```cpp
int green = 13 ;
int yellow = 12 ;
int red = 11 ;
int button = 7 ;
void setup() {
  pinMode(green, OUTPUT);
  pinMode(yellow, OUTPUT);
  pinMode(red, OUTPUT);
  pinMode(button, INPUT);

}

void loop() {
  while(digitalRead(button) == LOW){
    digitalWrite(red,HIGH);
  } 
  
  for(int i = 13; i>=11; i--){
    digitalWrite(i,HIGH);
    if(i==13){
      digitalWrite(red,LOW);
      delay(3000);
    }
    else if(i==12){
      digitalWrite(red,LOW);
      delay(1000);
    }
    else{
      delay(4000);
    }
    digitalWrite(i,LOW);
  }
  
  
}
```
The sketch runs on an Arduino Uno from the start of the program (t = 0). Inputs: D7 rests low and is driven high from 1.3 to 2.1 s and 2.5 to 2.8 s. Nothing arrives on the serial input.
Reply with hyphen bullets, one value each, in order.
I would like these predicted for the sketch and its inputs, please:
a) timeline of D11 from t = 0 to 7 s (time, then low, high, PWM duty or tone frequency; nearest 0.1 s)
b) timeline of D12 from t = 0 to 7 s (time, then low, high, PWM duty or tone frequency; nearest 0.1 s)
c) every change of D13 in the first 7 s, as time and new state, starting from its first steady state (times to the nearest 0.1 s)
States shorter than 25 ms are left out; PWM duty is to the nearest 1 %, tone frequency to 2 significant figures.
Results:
- 0 s high; 1.3 s low; 5.3 s high
- 0 s low; 4.3 s high; 5.3 s low
- 0 s low; 1.3 s high; 4.3 s low
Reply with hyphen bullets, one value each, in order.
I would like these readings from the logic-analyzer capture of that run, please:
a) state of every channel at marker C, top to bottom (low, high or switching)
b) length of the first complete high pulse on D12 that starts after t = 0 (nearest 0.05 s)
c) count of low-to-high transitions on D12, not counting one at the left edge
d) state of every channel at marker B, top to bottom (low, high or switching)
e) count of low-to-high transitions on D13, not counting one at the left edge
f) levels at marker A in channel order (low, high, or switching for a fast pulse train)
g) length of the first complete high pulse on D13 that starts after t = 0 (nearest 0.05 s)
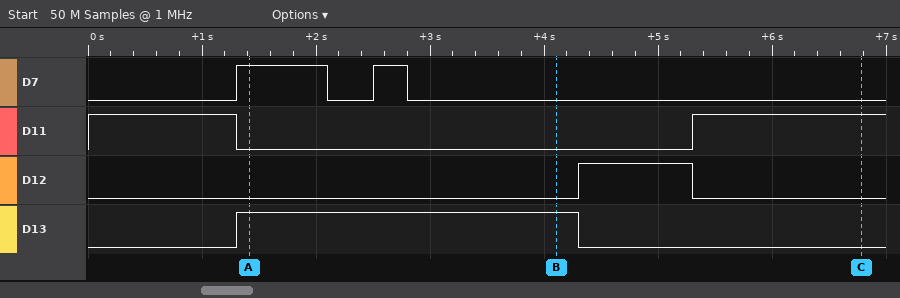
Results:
- D7 low, D11 high, D12 low, D13 low
- 1.00 s
- 1
- D7 low, D11 low, D12 low, D13 high
- 1
- D7 high, D11 low, D12 low, D13 high
- 3.00 s
